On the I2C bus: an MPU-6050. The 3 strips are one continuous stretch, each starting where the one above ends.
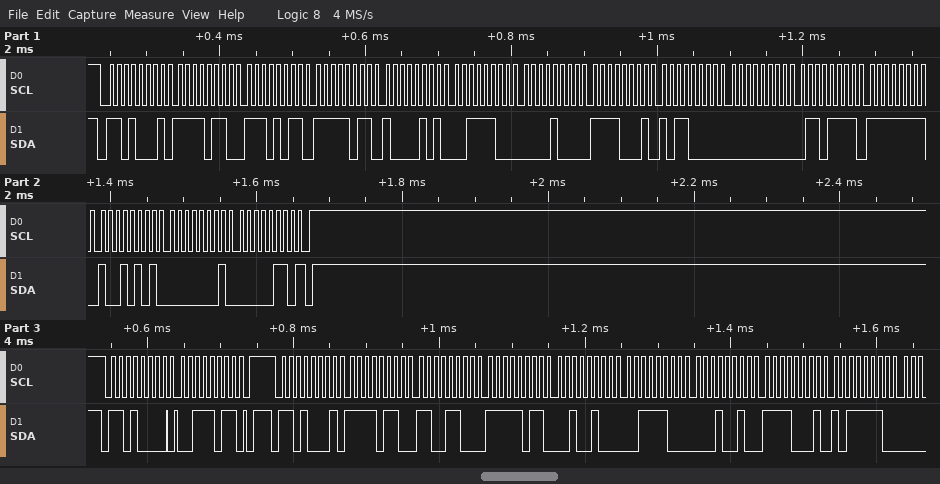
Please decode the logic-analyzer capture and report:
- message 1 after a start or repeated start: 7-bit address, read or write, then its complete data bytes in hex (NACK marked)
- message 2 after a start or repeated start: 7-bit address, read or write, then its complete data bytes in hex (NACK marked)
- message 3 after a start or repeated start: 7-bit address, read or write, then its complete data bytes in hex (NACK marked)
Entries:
0x68 read: F6 EB FB 85 3C 08 F1 B0 00 6F FF 95 01 06 NACK
0x68 write: 3B
0x68 read: F6 CC FB 24 3C 12 F1 BE
